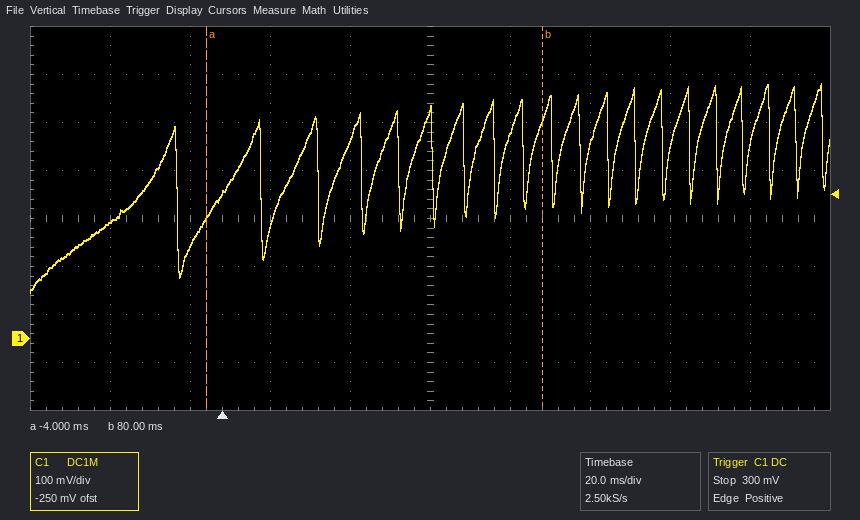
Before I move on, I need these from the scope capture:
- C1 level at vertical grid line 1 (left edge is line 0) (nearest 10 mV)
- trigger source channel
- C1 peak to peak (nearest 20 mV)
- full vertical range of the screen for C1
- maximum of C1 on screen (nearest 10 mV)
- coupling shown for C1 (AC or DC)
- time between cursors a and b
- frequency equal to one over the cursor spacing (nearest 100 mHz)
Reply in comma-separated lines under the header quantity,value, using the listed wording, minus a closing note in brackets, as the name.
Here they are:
quantity,value
C1 level at vertical grid line 1 (left edge is line 0),240 mV
trigger source channel,C1
C1 peak to peak,440 mV
full vertical range of the screen for C1,800 mV
maximum of C1 on screen,530 mV
coupling shown for C1,DC
time between cursors a and b,84 ms
frequency equal to one over the cursor spacing,11.9 Hz
